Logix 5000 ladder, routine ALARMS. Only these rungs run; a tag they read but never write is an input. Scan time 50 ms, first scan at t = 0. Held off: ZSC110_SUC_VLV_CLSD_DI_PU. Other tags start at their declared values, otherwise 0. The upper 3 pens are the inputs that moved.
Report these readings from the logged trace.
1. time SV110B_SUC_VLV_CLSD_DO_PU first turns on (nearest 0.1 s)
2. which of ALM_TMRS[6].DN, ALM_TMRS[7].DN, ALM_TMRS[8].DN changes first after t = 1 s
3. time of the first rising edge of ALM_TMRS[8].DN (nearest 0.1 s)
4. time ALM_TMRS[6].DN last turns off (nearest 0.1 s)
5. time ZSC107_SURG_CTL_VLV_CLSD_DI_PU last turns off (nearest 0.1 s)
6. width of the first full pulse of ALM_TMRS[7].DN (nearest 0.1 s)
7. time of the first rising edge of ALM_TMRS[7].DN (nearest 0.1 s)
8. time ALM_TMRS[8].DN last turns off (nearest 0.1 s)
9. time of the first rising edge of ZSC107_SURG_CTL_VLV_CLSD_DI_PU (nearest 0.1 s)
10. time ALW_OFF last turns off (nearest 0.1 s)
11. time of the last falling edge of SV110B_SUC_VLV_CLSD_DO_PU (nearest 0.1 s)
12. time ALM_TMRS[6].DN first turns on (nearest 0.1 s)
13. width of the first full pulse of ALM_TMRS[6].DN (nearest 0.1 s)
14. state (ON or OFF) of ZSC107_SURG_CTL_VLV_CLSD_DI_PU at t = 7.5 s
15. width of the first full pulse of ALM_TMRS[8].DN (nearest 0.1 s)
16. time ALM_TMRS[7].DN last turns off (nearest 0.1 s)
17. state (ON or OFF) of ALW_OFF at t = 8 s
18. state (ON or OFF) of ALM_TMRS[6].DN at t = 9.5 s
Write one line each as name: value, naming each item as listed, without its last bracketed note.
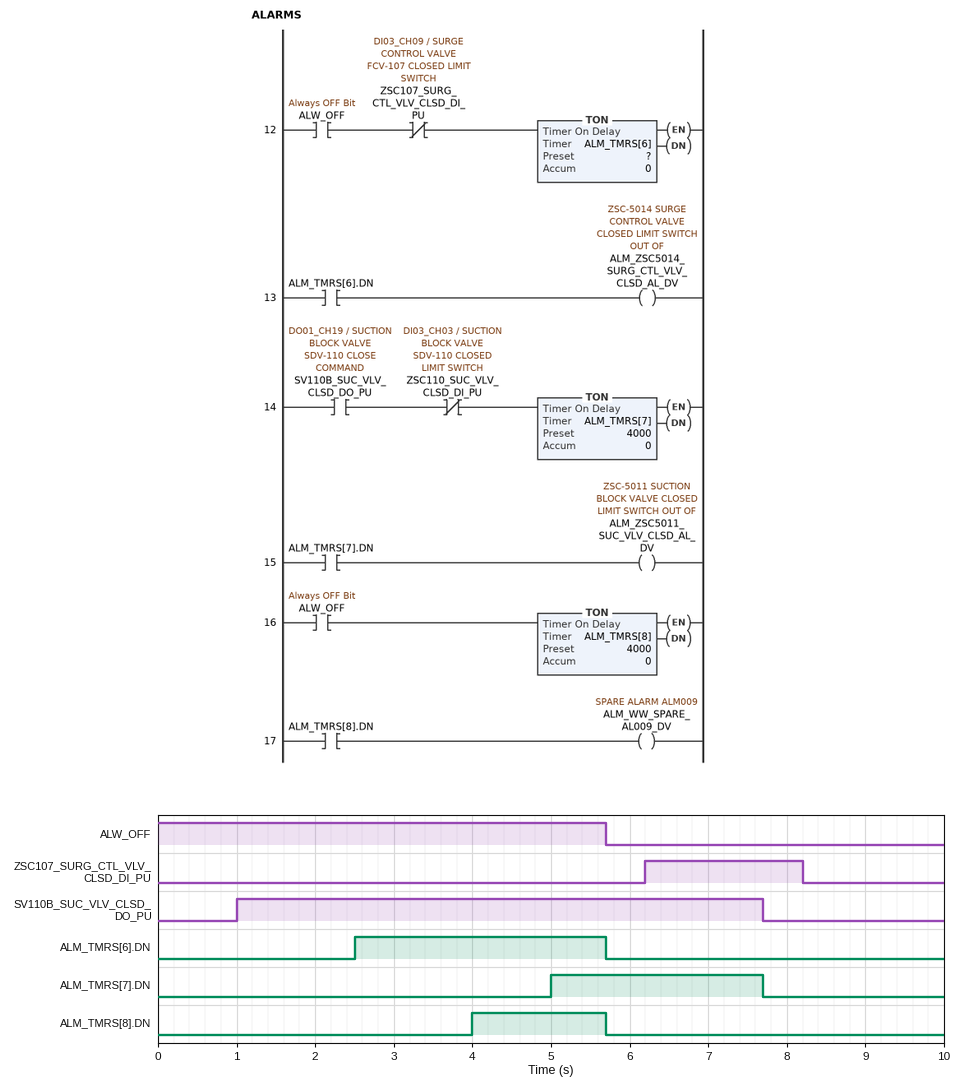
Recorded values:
time SV110B_SUC_VLV_CLSD_DO_PU first turns on: 1.0 s
which of ALM_TMRS[6].DN, ALM_TMRS[7].DN, ALM_TMRS[8].DN changes first after t = 1 s: ALM_TMRS[6].DN
time of the first rising edge of ALM_TMRS[8].DN: 4.0 s
time ALM_TMRS[6].DN last turns off: 5.7 s
time ZSC107_SURG_CTL_VLV_CLSD_DI_PU last turns off: 8.2 s
width of the first full pulse of ALM_TMRS[7].DN: 2.7 s
time of the first rising edge of ALM_TMRS[7].DN: 5.0 s
time ALM_TMRS[8].DN last turns off: 5.7 s
time of the first rising edge of ZSC107_SURG_CTL_VLV_CLSD_DI_PU: 6.2 s
time ALW_OFF last turns off: 5.7 s
time of the last falling edge of SV110B_SUC_VLV_CLSD_DO_PU: 7.7 s
time ALM_TMRS[6].DN first turns on: 2.5 s
width of the first full pulse of ALM_TMRS[6].DN: 3.2 s
state (ON or OFF) of ZSC107_SURG_CTL_VLV_CLSD_DI_PU at t = 7.5 s: ON
width of the first full pulse of ALM_TMRS[8].DN: 1.7 s
time ALM_TMRS[7].DN last turns off: 7.7 s
state (ON or OFF) of ALW_OFF at t = 8 s: OFF
state (ON or OFF) of ALM_TMRS[6].DN at t = 9.5 s: OFF
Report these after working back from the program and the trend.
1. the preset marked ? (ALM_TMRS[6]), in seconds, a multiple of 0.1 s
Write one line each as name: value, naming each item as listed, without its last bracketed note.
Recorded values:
the preset marked ? (ALM_TMRS[6]), in seconds, a multiple of 0.1 s: 2.5 s
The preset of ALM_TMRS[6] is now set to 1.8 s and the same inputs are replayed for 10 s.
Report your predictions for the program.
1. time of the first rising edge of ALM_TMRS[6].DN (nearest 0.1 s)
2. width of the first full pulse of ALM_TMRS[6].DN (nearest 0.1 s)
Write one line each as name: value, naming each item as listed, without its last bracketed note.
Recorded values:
time of the first rising edge of ALM_TMRS[6].DN: 1.8 s
width of the first full pulse of ALM_TMRS[6].DN: 3.9 s
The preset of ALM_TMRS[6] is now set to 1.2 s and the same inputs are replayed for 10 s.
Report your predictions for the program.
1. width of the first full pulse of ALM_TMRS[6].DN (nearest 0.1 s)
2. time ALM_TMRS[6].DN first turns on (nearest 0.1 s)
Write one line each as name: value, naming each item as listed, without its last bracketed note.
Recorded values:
width of the first full pulse of ALM_TMRS[6].DN: 4.5 s
time ALM_TMRS[6].DN first turns on: 1.2 s
